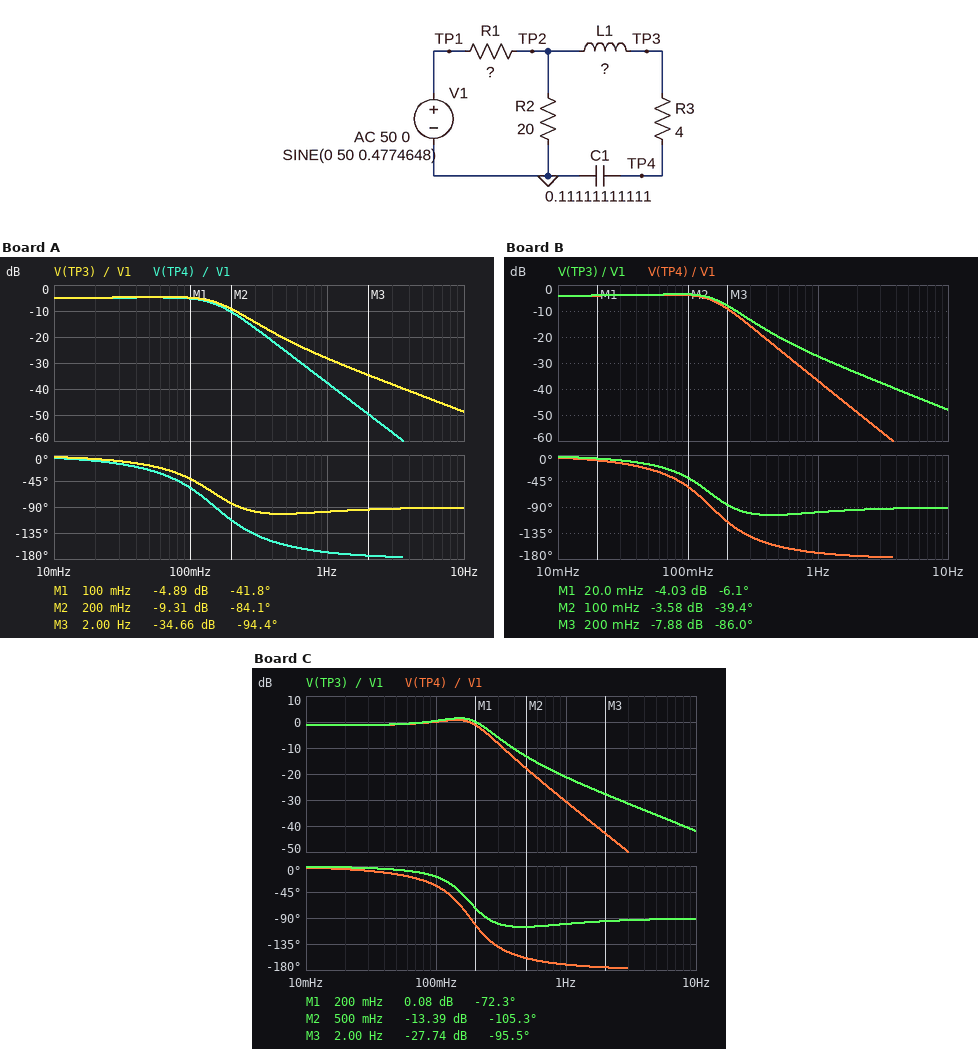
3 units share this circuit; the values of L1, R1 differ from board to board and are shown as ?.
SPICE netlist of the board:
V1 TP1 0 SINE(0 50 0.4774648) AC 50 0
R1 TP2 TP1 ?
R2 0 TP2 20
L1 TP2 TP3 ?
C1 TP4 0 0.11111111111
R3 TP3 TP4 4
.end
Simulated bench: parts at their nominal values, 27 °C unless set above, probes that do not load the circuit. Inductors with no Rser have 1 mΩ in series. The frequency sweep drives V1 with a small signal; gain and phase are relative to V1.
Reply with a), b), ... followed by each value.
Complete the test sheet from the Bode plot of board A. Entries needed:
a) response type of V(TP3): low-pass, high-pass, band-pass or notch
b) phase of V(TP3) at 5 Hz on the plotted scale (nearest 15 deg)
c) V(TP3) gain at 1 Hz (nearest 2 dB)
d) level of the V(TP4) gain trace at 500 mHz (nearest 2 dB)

a) low-pass
b) -90 deg
c) -28 dB
d) -26 dB
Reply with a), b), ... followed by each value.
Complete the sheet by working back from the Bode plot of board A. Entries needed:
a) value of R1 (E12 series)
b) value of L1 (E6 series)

a) 15 Ω
b) 10 H
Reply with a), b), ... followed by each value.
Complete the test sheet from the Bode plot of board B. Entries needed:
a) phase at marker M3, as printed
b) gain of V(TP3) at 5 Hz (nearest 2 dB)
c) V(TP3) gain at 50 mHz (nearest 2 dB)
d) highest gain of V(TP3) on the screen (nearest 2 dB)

a) -86.0 deg
b) -42 dB
c) -4 dB
d) -4 dB
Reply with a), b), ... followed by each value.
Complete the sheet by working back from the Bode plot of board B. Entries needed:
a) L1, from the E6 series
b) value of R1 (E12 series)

a) 10 H
b) 12 Ω
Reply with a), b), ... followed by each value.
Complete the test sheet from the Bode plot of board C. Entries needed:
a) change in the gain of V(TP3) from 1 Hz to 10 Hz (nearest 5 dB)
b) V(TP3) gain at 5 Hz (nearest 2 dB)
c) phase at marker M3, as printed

a) -20 dB
b) -36 dB
c) -95.5 deg
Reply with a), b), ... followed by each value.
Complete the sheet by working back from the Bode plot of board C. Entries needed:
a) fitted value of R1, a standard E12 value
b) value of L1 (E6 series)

a) 3.3 Ω
b) 6.8 H
